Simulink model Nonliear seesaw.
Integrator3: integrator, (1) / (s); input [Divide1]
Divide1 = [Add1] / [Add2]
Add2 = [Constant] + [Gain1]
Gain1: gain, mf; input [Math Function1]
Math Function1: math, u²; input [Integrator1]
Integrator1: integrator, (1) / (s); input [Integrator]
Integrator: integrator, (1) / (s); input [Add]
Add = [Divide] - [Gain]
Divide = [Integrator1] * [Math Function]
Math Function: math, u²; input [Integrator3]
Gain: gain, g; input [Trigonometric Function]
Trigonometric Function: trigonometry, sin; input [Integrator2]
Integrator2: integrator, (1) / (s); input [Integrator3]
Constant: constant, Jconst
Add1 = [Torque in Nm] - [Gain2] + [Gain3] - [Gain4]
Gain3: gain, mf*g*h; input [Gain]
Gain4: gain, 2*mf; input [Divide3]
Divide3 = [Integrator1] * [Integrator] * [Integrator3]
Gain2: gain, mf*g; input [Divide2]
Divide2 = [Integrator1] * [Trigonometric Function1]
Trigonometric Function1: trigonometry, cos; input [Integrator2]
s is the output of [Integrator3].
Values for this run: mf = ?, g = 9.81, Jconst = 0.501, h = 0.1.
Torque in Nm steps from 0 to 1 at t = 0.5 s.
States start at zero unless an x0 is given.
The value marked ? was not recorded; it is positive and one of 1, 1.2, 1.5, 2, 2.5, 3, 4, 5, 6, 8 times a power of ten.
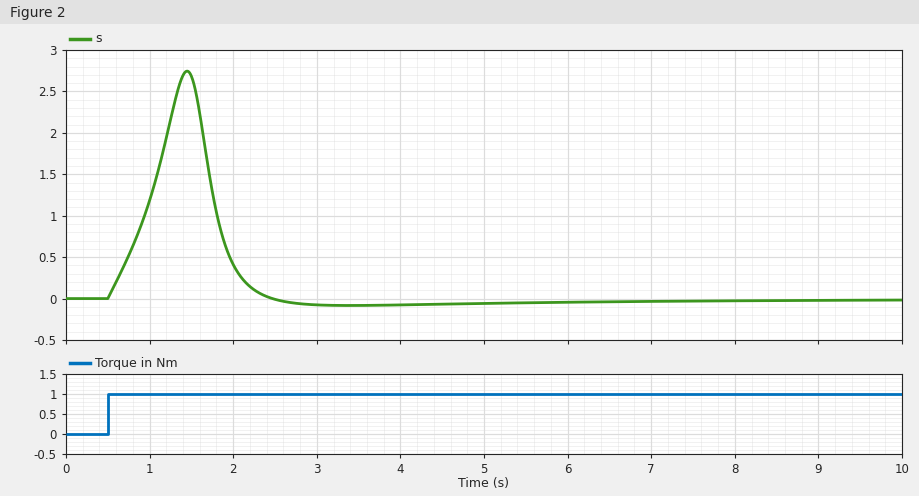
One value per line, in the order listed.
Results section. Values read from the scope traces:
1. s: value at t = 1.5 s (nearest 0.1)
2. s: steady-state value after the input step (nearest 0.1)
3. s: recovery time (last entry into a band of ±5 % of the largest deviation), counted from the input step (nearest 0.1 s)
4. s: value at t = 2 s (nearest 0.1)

2.7
0.0
1.7 s
0.4
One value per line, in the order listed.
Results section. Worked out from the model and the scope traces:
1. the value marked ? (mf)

0.2
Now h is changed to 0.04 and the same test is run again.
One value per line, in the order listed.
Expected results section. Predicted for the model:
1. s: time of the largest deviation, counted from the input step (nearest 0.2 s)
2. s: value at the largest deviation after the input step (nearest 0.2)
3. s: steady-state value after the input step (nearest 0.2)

1.0 s
2.2
0.0
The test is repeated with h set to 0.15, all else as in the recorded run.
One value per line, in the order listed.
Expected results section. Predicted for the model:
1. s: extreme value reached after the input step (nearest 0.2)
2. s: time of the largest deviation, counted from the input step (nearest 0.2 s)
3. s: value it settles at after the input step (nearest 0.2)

3.2
1.0 s
0.0
